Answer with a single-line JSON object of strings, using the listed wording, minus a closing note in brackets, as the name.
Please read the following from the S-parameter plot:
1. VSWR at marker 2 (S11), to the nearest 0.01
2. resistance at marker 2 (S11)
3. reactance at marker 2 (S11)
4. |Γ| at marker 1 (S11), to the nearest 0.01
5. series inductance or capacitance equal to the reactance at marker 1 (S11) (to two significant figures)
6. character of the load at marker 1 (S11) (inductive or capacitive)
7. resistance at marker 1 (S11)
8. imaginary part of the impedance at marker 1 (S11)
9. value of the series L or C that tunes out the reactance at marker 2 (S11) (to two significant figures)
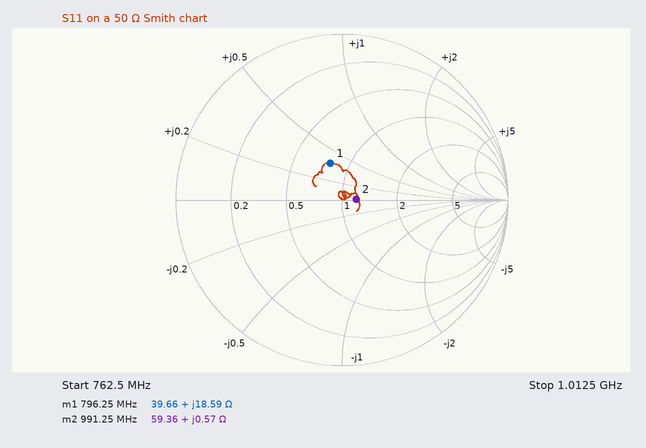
{"VSWR at marker 2 (S11), to the nearest 0.01": "1.19", "resistance at marker 2": "59.36 Ω", "reactance at marker 2": "+0.57 Ω", "|Γ| at marker 1 (S11), to the nearest 0.01": "0.23", "series inductance or capacitance equal to the reactance at marker 1 (S11)": "3.7 nH", "character of the load at marker 1 (S11)": "inductive", "resistance at marker 1": "39.66 Ω", "imaginary part of the impedance at marker 1": "+18.59 Ω", "value of the series L or C that tunes out the reactance at marker 2 (S11)": "280 pF"}
